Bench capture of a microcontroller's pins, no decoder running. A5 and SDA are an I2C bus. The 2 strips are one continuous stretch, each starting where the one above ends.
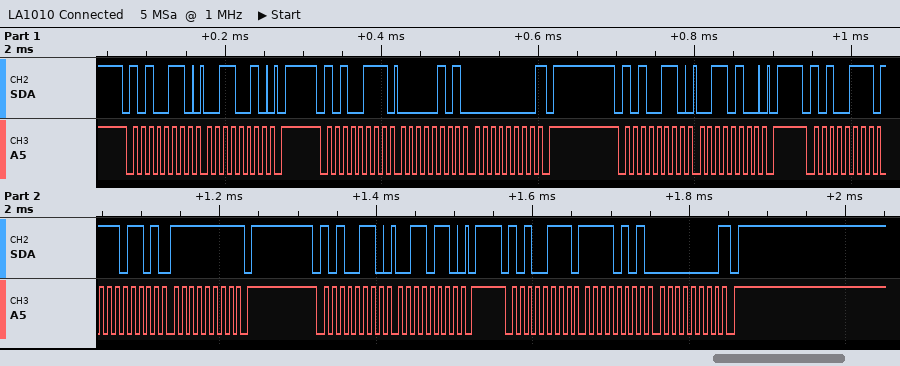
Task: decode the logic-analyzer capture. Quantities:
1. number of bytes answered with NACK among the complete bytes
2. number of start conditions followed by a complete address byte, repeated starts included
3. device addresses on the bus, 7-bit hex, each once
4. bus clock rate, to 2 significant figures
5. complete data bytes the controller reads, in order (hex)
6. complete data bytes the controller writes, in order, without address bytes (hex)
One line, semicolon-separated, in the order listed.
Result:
3; 6; 0x53; 100 kHz; 05 00 ED FF F5 00; 32 34 36
